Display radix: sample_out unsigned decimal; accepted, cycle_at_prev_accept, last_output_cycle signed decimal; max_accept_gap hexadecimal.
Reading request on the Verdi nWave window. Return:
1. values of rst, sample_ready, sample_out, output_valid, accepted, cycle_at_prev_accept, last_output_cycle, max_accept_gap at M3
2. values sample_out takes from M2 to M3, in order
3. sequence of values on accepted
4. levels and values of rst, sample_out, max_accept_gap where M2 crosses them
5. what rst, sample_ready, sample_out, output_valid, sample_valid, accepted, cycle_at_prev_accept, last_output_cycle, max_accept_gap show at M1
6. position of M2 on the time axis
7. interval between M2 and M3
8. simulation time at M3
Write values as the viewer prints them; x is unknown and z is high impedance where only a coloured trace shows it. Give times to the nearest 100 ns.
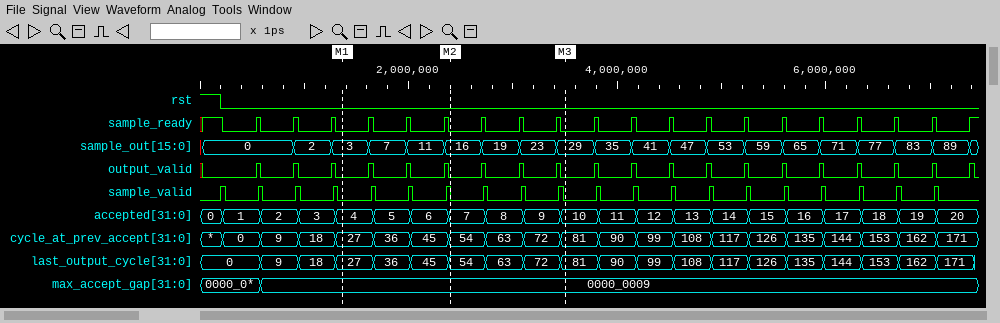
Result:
rst=0, sample_ready=0, sample_out=29, output_valid=0, accepted=10, cycle_at_prev_accept=81, last_output_cycle=81, max_accept_gap=0000_0009
16, 19, 23, 29
0, 1, 2, 3, 4, 5, 6, 7, 8, 9, 10, 11, 12, 13, 14, 15, 16, 17, 18, 19, 20
rst=0, sample_out=16, max_accept_gap=0000_0009
rst=0, sample_ready=0, sample_out=3, output_valid=0, sample_valid=0, accepted=4, cycle_at_prev_accept=27, last_output_cycle=27, max_accept_gap=0000_0009
2400 ns
1100 ns
3500 ns
